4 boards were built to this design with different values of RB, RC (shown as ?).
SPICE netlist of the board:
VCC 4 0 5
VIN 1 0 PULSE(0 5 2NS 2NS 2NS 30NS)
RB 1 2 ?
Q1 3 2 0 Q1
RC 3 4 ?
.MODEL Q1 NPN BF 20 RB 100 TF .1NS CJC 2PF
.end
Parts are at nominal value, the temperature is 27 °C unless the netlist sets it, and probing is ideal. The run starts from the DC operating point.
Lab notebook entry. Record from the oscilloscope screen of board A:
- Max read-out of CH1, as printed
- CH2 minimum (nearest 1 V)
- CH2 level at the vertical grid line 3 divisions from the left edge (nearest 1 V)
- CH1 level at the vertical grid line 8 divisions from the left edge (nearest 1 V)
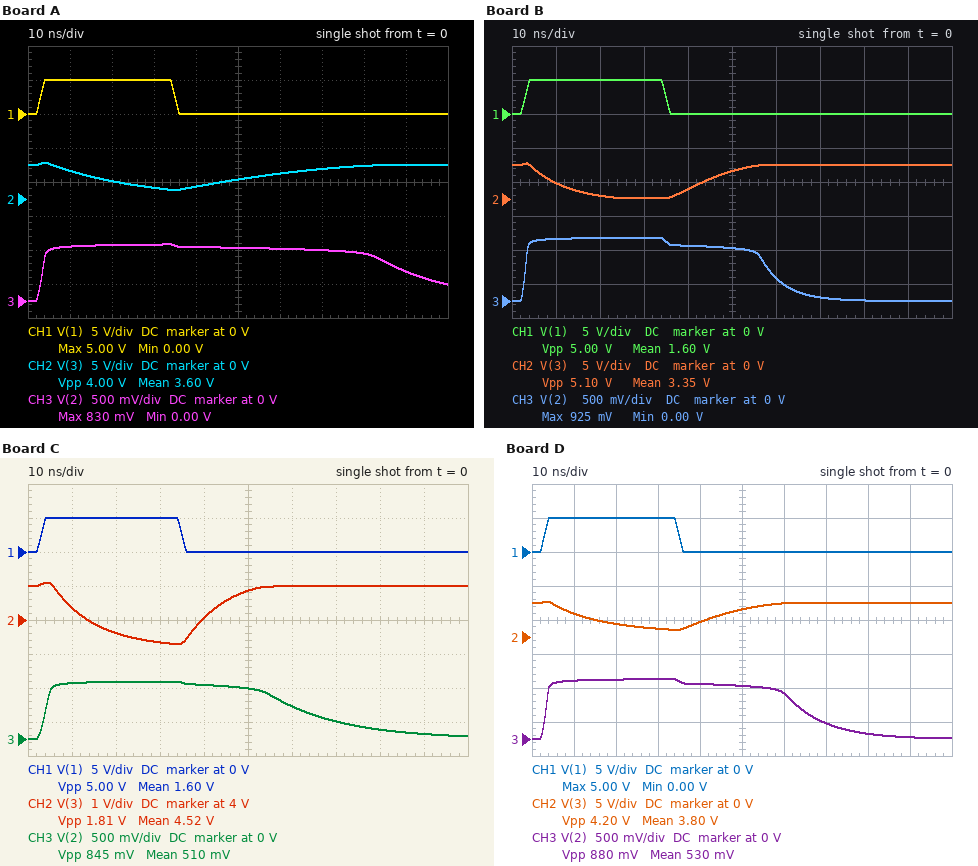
5.00 V
1 V
2 V
0 V
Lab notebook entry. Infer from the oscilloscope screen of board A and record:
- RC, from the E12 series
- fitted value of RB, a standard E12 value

1.2 kΩ
15 kΩ
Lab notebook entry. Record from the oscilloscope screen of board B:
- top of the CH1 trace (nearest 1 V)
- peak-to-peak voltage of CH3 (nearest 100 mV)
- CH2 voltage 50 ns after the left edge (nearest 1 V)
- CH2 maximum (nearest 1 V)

5 V
900 mV
4 V
5 V
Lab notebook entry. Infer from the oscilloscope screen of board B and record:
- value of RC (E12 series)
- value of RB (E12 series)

390 Ω
4.7 kΩ
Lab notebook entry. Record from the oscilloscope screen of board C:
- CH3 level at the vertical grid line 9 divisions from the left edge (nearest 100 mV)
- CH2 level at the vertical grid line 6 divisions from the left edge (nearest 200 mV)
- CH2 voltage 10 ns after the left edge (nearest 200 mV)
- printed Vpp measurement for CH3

100 mV
5.0 V
4.4 V
845 mV
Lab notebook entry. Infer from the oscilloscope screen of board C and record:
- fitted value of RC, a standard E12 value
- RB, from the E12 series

330 Ω
15 kΩ
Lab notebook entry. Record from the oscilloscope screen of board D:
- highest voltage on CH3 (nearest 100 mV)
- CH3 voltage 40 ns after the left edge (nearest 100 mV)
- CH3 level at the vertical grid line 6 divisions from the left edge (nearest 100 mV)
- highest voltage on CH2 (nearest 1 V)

900 mV
800 mV
700 mV
5 V
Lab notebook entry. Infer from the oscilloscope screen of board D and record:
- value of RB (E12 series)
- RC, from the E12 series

8.2 kΩ
470 Ω
